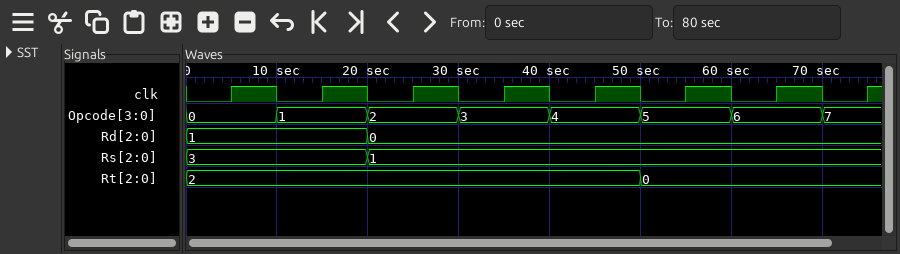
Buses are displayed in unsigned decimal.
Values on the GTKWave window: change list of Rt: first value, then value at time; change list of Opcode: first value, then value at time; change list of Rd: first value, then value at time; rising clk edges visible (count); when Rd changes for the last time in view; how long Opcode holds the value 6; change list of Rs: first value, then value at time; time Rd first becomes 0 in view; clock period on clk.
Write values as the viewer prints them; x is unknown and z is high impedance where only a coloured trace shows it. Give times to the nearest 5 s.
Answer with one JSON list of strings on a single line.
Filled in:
["2, 0 at 50 s", "0, 1 at 10 s, 2 at 20 s, 3 at 30 s, 4 at 40 s, 5 at 50 s, 6 at 60 s, 7 at 70 s", "1, 0 at 20 s", "8", "20 s", "10 s", "3, 1 at 20 s", "20 s", "10 s"]
